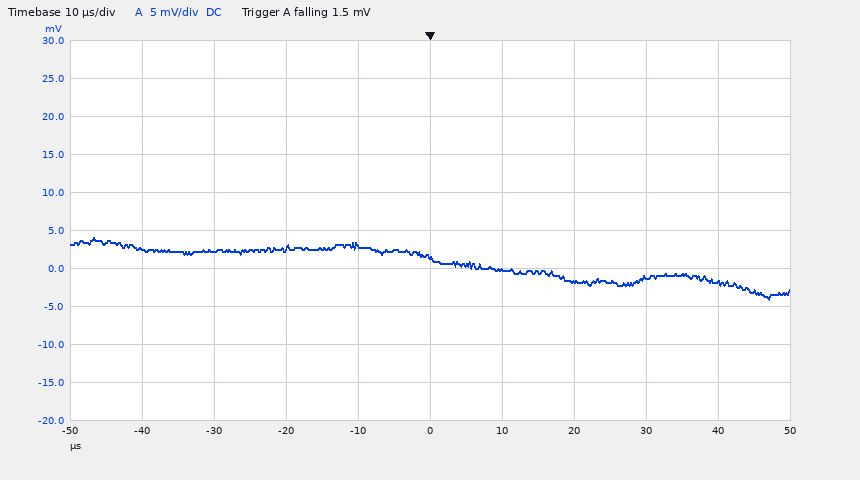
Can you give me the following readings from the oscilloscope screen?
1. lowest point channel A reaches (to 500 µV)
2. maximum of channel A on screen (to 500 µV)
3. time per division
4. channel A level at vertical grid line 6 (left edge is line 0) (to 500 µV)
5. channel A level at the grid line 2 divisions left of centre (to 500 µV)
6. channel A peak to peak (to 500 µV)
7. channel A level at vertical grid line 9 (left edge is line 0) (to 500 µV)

-4.0 mV
4.0 mV
10 µs
0.0 mV
2.5 mV
8.0 mV
-2.0 mV
